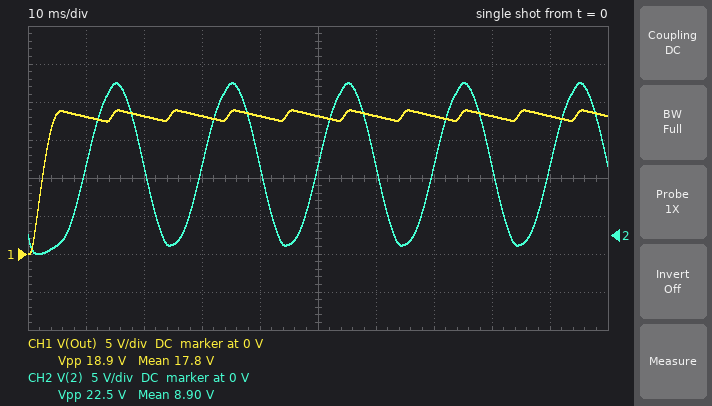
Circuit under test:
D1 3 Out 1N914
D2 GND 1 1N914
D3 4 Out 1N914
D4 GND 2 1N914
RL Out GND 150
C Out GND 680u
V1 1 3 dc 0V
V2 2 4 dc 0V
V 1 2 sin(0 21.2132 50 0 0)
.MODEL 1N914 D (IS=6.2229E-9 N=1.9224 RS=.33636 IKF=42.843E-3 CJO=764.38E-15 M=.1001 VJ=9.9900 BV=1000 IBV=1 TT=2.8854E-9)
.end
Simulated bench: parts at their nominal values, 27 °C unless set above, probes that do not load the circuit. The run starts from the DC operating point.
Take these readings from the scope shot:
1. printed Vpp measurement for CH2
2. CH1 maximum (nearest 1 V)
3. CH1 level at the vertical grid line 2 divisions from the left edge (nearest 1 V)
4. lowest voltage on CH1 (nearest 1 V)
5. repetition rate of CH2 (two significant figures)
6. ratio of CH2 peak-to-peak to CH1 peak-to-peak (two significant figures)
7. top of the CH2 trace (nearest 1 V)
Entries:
22.5 V
19 V
18 V
0 V
50 Hz
1.2
20 V
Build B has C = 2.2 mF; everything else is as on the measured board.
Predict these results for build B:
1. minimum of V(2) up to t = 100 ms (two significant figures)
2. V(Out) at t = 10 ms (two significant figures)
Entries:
-4.5 V
17 V
